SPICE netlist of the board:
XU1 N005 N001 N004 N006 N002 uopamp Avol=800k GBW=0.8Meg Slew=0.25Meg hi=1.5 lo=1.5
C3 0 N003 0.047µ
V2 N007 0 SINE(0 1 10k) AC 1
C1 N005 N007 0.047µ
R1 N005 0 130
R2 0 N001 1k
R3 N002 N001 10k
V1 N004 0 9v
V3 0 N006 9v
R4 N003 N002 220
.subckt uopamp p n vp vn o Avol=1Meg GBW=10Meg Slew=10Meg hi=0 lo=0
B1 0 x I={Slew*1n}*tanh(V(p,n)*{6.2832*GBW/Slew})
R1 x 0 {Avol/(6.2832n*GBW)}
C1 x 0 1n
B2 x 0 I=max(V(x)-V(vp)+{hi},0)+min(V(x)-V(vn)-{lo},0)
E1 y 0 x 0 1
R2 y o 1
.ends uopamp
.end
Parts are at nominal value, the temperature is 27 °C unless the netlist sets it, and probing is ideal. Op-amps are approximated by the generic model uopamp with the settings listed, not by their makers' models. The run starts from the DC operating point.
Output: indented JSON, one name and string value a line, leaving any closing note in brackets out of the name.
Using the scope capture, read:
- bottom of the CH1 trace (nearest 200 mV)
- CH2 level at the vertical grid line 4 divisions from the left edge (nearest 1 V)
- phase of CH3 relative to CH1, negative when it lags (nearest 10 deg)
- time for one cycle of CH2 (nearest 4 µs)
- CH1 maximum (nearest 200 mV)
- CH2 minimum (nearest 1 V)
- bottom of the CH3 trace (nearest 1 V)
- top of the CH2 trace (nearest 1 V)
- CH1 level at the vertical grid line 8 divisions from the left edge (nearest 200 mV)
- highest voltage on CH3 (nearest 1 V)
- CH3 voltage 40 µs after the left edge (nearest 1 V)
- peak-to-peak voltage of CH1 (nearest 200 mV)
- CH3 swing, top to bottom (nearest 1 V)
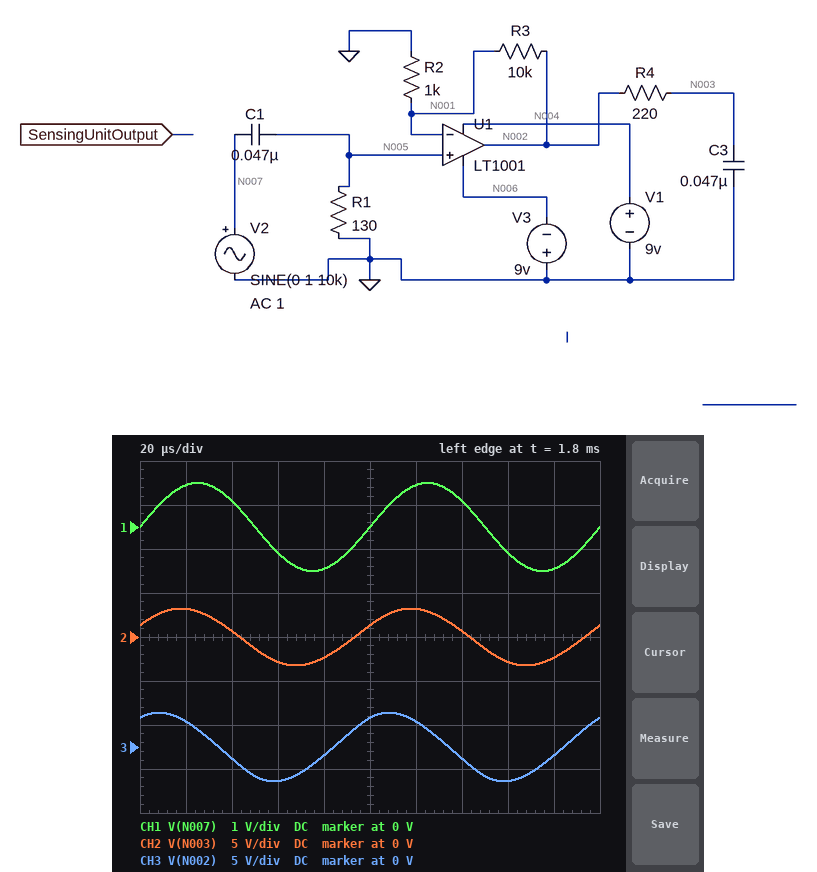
{
  "bottom of the CH1 trace": "-1.0 V",
  "CH2 level at the vertical grid line 4 divisions from the left edge": "-2 V",
  "phase of CH3 relative to CH1, negative when it lags": "60 deg",
  "time for one cycle of CH2": "100 µs",
  "CH1 maximum": "1.0 V",
  "CH2 minimum": "-3 V",
  "bottom of the CH3 trace": "-4 V",
  "top of the CH2 trace": "3 V",
  "CH1 level at the vertical grid line 8 divisions from the left edge": "-600 mV",
  "highest voltage on CH3": "4 V",
  "CH3 voltage 40 µs after the left edge": "-1 V",
  "peak-to-peak voltage of CH1": "2.0 V",
  "CH3 swing, top to bottom": "8 V"
}
